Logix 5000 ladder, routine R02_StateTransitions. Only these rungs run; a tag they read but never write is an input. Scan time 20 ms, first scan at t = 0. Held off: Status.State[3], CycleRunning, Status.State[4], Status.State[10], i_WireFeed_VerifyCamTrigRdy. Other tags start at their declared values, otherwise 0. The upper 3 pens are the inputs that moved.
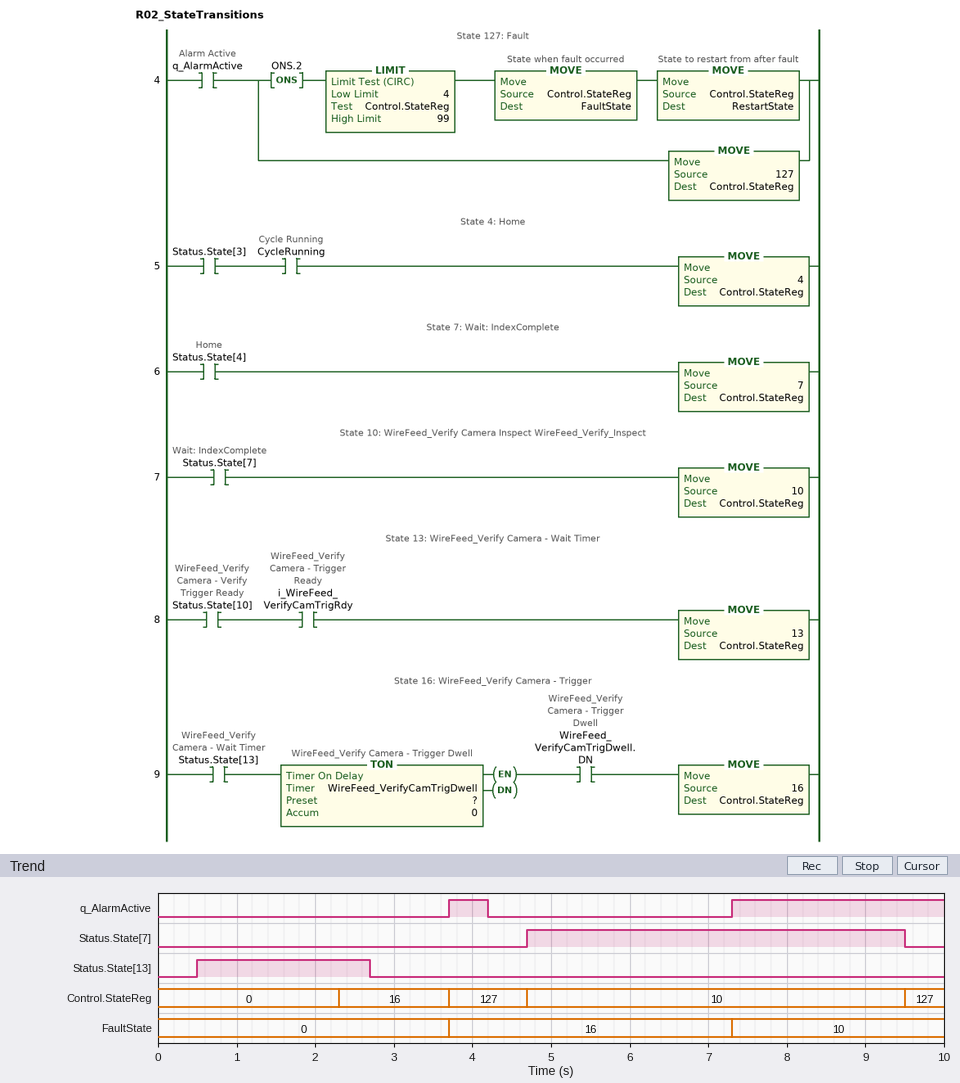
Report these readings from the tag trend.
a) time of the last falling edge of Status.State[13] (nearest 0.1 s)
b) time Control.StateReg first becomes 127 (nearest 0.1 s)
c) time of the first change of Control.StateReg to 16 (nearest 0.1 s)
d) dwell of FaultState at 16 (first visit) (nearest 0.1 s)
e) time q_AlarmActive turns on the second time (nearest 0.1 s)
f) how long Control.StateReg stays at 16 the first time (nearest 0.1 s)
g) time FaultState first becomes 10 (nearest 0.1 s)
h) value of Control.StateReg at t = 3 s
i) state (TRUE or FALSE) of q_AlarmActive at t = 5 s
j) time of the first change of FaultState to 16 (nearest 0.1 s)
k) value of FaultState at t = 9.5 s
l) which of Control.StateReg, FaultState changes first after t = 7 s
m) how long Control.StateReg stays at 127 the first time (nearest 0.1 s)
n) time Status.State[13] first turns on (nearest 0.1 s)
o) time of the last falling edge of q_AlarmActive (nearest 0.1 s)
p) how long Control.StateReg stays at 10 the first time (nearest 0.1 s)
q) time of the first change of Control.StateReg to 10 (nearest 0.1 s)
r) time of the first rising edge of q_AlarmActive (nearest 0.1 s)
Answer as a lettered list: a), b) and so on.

a) 2.7 s
b) 3.7 s
c) 2.3 s
d) 3.6 s
e) 7.3 s
f) 1.4 s
g) 7.3 s
h) 16
i) FALSE
j) 3.7 s
k) 10
l) FaultState
m) 1.0 s
n) 0.5 s
o) 4.2 s
p) 4.8 s
q) 4.7 s
r) 3.7 s
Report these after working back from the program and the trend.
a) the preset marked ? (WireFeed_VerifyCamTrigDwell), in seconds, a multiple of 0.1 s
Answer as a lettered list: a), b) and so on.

a) 1.8 s
